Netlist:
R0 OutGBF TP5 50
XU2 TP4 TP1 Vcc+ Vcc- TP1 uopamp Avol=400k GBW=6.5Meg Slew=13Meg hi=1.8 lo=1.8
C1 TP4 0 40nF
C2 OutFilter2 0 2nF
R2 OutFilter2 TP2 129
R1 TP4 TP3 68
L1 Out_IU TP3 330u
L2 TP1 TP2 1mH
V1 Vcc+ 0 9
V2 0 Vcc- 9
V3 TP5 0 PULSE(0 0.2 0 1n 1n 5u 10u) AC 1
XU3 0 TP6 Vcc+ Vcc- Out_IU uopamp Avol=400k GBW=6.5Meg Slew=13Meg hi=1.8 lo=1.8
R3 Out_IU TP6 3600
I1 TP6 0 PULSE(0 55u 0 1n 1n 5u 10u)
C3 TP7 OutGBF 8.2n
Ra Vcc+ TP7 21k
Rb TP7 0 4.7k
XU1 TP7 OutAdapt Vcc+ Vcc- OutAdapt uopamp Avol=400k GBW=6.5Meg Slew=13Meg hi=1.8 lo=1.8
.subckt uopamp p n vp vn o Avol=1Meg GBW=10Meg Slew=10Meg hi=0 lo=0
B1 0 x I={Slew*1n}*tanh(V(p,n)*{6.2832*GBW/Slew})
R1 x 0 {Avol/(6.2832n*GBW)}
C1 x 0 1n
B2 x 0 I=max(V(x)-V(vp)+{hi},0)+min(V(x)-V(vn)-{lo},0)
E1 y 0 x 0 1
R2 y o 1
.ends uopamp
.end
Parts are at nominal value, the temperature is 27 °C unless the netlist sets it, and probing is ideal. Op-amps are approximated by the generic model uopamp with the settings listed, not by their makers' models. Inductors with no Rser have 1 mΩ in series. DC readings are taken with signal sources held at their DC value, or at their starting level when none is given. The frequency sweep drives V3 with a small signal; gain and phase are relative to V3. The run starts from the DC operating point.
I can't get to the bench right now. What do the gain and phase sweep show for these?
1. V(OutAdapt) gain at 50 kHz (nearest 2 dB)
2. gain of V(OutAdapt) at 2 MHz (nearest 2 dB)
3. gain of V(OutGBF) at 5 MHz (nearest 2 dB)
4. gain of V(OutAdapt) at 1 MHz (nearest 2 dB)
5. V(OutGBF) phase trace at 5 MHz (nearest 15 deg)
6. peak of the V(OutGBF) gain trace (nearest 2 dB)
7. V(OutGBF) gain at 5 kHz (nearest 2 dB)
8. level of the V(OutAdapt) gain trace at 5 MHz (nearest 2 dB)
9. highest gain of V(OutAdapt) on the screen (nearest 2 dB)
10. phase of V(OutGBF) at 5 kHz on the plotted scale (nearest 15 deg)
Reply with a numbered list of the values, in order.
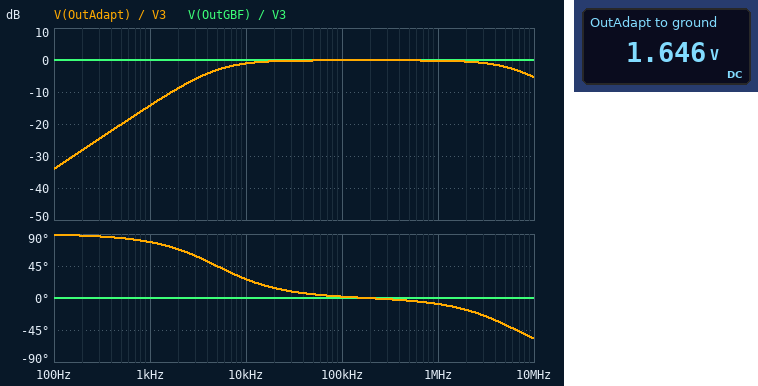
1. 0 dB
2. 0 dB
3. 0 dB
4. 0 dB
5. 0 deg
6. 0 dB
7. 0 dB
8. -2 dB
9. 0 dB
10. 0 deg
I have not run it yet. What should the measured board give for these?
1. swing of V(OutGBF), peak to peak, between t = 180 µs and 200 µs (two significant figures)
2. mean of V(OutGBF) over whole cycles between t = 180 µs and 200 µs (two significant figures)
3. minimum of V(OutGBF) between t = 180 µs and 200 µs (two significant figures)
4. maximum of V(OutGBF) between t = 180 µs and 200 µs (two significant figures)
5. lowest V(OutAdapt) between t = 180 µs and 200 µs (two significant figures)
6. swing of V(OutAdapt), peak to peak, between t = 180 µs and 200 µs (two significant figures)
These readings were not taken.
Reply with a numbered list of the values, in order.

1. 200 mV
2. 100 mV
3. 1.2 mV
4. 200 mV
5. 1.5 V
6. 210 mV
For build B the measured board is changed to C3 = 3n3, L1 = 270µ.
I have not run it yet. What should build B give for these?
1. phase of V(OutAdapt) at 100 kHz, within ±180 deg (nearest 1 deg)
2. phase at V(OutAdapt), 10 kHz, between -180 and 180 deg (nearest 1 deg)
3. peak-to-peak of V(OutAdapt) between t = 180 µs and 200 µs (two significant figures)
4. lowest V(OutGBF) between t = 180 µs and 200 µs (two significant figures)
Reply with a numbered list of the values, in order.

1. 6 deg
2. 51 deg
3. 230 mV
4. 1.0 mV
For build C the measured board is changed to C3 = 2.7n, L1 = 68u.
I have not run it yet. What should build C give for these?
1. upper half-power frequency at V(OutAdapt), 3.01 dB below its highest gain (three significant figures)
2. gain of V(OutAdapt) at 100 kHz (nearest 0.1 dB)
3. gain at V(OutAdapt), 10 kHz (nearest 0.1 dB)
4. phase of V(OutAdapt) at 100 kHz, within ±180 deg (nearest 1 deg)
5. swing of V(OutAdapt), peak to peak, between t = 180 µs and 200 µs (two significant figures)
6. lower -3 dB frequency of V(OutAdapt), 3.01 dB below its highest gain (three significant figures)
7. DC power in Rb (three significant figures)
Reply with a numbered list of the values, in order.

1. 6.53 MHz
2. -0.2 dB
3. -5.3 dB
4. 8 deg
5. 240 mV
6. 15.1 kHz
7. 576 µW
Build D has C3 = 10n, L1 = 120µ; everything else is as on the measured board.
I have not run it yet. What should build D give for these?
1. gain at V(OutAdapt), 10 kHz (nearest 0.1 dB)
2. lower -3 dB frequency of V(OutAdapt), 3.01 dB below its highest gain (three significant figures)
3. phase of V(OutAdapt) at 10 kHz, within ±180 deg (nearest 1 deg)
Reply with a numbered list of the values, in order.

1. -0.8 dB
2. 4.09 kHz
3. 22 deg
